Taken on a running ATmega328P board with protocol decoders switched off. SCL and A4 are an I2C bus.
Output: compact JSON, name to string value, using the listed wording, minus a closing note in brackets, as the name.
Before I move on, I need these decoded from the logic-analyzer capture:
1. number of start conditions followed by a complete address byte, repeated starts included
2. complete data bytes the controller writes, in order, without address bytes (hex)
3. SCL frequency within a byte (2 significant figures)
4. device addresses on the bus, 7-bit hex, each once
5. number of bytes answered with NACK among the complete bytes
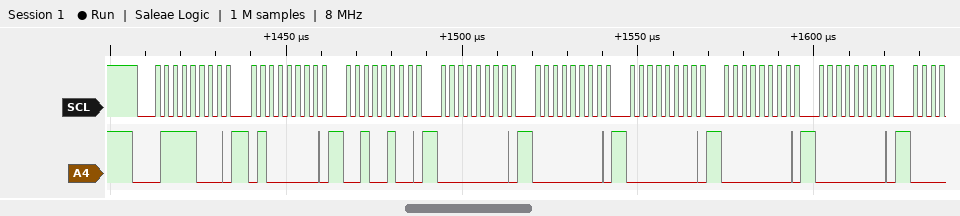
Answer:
{"number of start conditions followed by a complete address byte, repeated starts included": "1", "complete data bytes the controller writes, in order, without address bytes": "40 24 00 00 00 00 00", "SCL frequency within a byte": "400 kHz", "device addresses on the bus, 7-bit hex, each once": "0x3C", "number of bytes answered with NACK among the complete bytes": "0"}
